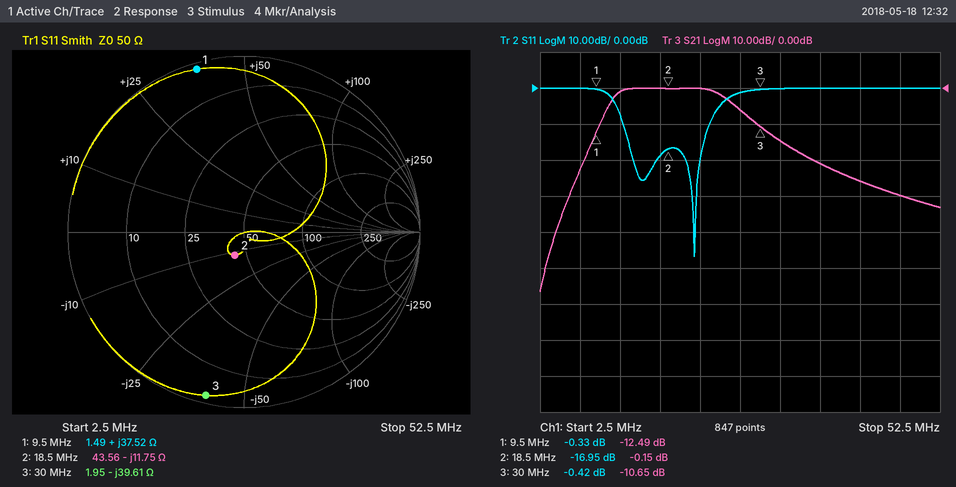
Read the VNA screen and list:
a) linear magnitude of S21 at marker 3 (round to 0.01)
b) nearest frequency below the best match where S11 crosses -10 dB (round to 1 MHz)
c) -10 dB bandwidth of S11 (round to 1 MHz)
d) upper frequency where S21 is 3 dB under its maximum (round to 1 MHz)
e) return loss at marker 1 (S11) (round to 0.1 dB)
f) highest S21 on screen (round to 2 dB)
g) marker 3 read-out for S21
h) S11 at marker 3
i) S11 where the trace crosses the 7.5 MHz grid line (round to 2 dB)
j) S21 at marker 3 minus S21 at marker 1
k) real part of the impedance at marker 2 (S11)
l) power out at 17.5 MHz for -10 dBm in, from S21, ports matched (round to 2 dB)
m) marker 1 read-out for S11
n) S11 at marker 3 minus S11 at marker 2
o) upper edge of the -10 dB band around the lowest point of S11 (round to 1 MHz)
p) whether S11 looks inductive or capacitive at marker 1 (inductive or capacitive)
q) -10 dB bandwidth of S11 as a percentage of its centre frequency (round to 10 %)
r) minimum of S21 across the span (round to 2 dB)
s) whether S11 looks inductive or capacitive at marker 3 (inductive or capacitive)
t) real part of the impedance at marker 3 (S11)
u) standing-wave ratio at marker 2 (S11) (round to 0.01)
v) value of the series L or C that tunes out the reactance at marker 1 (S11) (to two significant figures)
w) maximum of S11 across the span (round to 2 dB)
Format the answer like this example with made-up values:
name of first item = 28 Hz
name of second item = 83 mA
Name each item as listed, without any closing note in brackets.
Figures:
linear magnitude of S21 at marker 3 = 0.29
nearest frequency below the best match where S11 crosses -10 dB = 13 MHz
-10 dB bandwidth of S11 = 11 MHz
upper frequency where S21 is 3 dB under its maximum = 26 MHz
return loss at marker 1 (S11) = 0.3 dB
highest S21 on screen = 0 dB
marker 3 read-out for S21 = -10.65 dB
S11 at marker 3 = -0.42 dB
S11 where the trace crosses the 7.5 MHz grid line = 0 dB
S21 at marker 3 minus S21 at marker 1 = 1.84 dB
real part of the impedance at marker 2 = 43.56 Ω
power out at 17.5 MHz for -10 dBm in, from S21, ports matched = -10 dBm
marker 1 read-out for S11 = -0.33 dB
S11 at marker 3 minus S11 at marker 2 = 16.53 dB
upper edge of the -10 dB band around the lowest point of S11 = 24 MHz
whether S11 looks inductive or capacitive at marker 1 = inductive
-10 dB bandwidth of S11 as a percentage of its centre frequency = 60 %
minimum of S21 across the span = -56 dB
whether S11 looks inductive or capacitive at marker 3 = capacitive
real part of the impedance at marker 3 = 1.95 Ω
standing-wave ratio at marker 2 (S11) = 1.33
value of the series L or C that tunes out the reactance at marker 1 (S11) = 450 pF
maximum of S11 across the span = 0 dB
